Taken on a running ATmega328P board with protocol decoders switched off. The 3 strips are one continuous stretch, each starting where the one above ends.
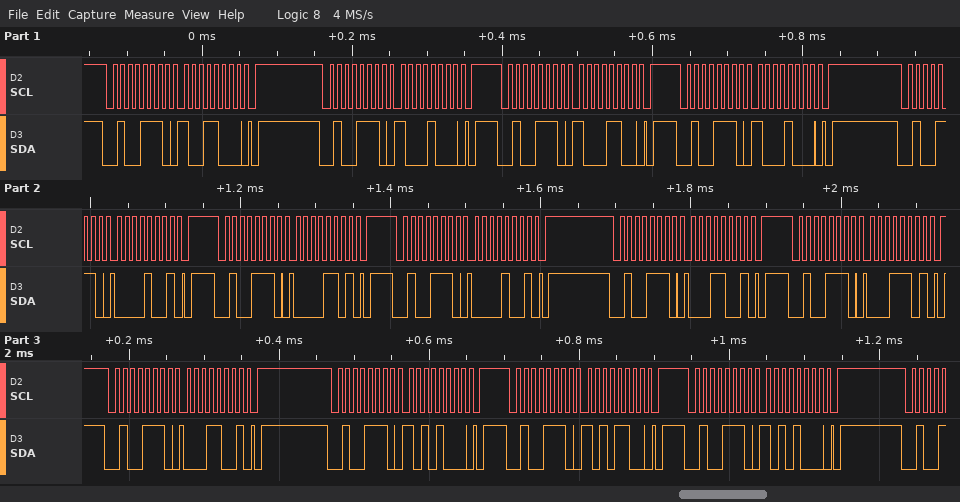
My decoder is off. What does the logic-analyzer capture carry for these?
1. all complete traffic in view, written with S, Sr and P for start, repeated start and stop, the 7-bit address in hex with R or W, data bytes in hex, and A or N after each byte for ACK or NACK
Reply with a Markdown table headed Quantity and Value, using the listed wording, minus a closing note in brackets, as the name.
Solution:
| Quantity | Value |
|---|---|
| all complete traffic in view, written with S, Sr and P for start, repeated start and stop, the 7-bit address in hex with R or W, data bytes in hex, and A or N after each byte for ACK or NACK | S 27W A 98 A P S 27W A 88 A P S 27W A 8C A P S 27W A 88 A P S 27W A 09 A P S 27W A 0D A P S 27W A 09 A P S 27W A 19 A P S 27W A 1D A P S 27W A 19 A P S 27W A A8 A P S 27W A AC A P S 27W A A8 A P |
